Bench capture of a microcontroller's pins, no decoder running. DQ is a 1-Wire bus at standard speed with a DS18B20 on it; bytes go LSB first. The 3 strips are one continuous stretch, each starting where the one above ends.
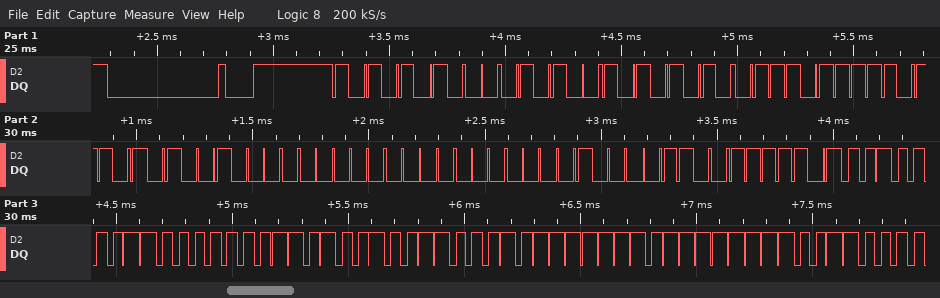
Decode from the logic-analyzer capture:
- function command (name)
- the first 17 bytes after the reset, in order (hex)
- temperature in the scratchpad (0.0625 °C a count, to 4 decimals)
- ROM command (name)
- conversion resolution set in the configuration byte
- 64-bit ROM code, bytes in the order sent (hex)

Read Scratchpad
55 28 55 EE 5B 09 00 00 61 BE 84 01 4B 46 7F FF 0C
24.2500 °C
Match ROM
12 bits
28 55 EE 5B 09 00 00 61
